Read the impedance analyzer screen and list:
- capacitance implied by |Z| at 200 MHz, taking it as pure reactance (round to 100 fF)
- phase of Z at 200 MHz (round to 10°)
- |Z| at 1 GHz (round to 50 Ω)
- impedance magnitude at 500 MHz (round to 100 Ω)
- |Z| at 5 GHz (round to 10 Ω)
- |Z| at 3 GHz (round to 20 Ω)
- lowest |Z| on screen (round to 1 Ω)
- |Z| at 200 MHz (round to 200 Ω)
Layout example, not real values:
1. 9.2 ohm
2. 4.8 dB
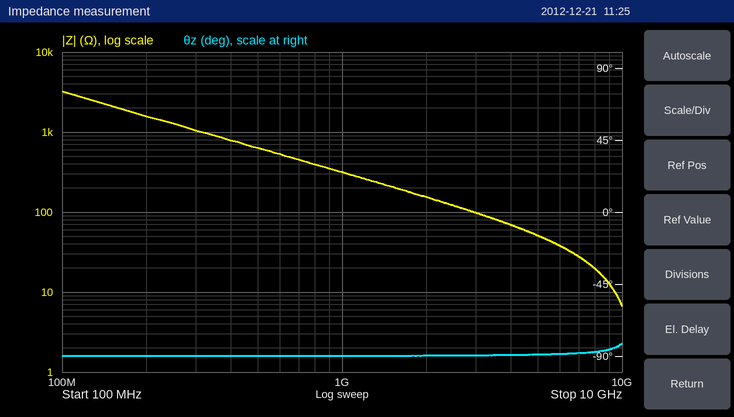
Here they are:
1. 500 fF
2. -90°
3. 300 Ω
4. 600 Ω
5. 50 Ω
6. 100 Ω
7. 7 Ω
8. 1.6 kΩ
